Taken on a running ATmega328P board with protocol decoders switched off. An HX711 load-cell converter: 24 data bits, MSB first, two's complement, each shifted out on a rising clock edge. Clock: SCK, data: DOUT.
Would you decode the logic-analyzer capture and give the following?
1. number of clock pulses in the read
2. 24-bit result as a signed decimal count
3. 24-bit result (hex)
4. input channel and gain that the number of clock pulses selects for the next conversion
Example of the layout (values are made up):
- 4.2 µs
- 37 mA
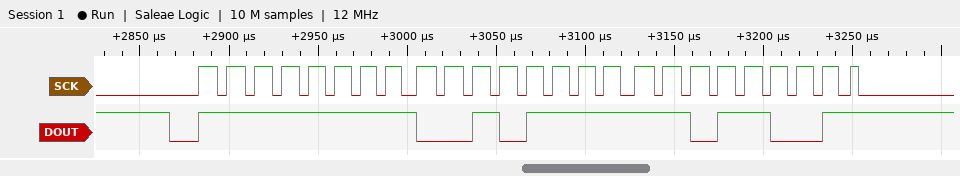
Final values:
- 25
- -53287
- 0xFF2FD9
- channel A, gain 128
